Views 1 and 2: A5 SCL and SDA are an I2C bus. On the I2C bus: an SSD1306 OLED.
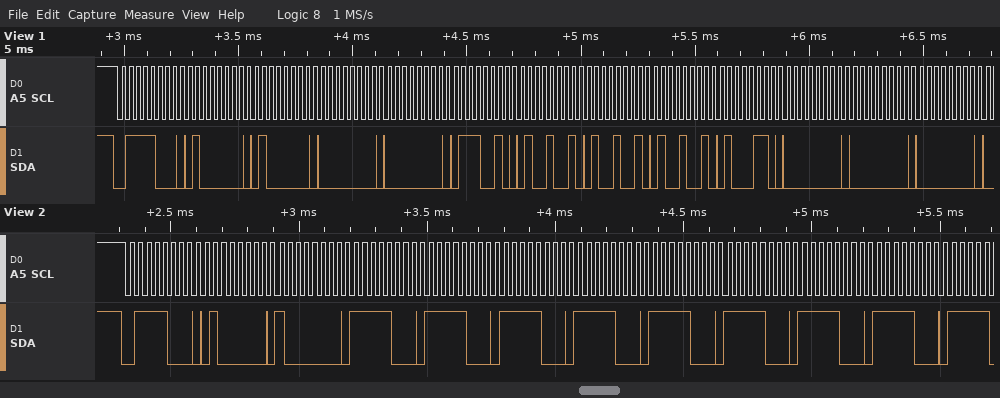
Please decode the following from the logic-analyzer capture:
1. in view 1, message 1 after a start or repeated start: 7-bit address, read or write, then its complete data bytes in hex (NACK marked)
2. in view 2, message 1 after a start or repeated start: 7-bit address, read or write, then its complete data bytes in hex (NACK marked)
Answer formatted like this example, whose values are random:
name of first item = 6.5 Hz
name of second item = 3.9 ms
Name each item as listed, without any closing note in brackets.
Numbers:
in view 1, message 1 after a start or repeated start: 7-bit address, read or write, then its complete data bytes in hex = 0x3C write: 40 40 00 00 72 49 49 49 46 00 00 00
in view 2, message 1 after a start or repeated start: 7-bit address, read or write, then its complete data bytes in hex = 0x3C write: 40 80 F8 F8 F8 F8 F8 F8 F8 F8
